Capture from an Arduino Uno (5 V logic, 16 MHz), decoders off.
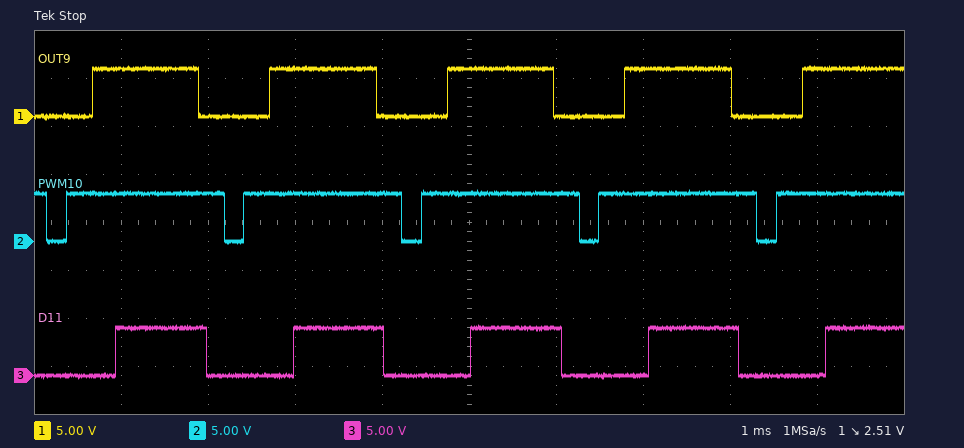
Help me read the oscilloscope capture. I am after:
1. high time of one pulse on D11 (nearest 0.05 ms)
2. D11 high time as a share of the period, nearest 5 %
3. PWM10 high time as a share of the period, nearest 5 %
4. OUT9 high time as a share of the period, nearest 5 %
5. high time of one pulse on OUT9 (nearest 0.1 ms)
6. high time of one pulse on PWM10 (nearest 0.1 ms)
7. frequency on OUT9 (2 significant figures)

1.05 ms
50 %
90 %
60 %
1.2 ms
1.8 ms
490 Hz
